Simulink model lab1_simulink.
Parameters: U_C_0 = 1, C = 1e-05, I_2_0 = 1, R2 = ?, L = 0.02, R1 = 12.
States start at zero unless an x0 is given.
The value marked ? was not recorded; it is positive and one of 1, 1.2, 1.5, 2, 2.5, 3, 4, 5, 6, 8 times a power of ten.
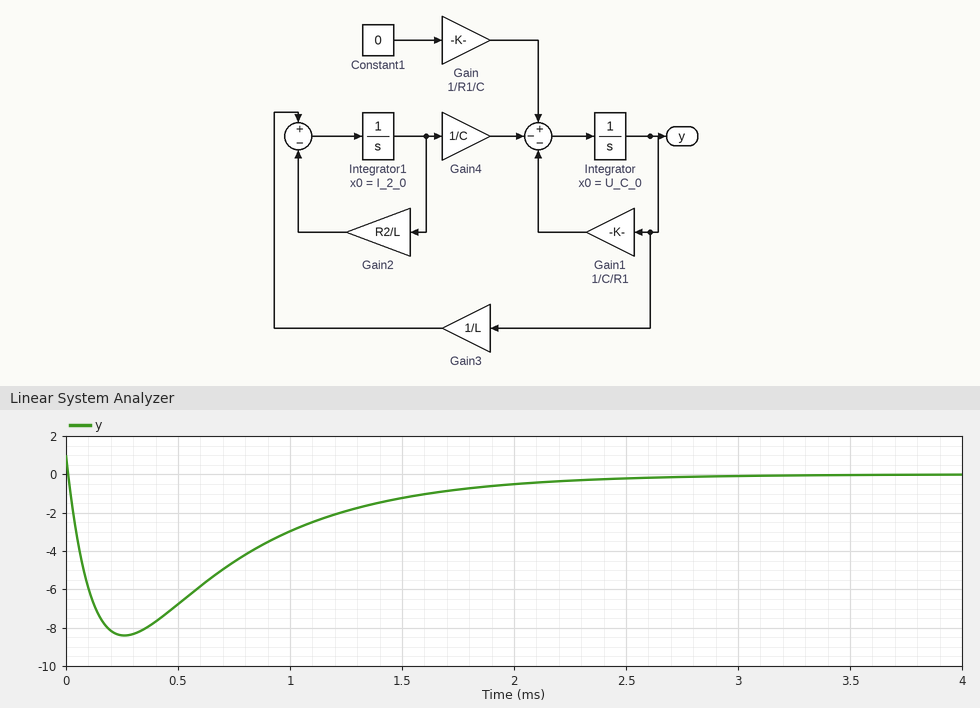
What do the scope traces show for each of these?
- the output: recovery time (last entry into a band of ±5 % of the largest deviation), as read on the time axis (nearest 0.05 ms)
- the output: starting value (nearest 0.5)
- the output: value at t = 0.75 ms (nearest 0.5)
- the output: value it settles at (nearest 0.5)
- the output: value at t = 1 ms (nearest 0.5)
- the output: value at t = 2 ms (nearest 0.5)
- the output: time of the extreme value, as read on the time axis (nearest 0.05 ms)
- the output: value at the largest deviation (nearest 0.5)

2.05 ms
1.0
-4.5
0.0
-3.0
-0.5
0.25 ms
-8.5
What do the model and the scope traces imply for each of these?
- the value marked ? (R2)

20
